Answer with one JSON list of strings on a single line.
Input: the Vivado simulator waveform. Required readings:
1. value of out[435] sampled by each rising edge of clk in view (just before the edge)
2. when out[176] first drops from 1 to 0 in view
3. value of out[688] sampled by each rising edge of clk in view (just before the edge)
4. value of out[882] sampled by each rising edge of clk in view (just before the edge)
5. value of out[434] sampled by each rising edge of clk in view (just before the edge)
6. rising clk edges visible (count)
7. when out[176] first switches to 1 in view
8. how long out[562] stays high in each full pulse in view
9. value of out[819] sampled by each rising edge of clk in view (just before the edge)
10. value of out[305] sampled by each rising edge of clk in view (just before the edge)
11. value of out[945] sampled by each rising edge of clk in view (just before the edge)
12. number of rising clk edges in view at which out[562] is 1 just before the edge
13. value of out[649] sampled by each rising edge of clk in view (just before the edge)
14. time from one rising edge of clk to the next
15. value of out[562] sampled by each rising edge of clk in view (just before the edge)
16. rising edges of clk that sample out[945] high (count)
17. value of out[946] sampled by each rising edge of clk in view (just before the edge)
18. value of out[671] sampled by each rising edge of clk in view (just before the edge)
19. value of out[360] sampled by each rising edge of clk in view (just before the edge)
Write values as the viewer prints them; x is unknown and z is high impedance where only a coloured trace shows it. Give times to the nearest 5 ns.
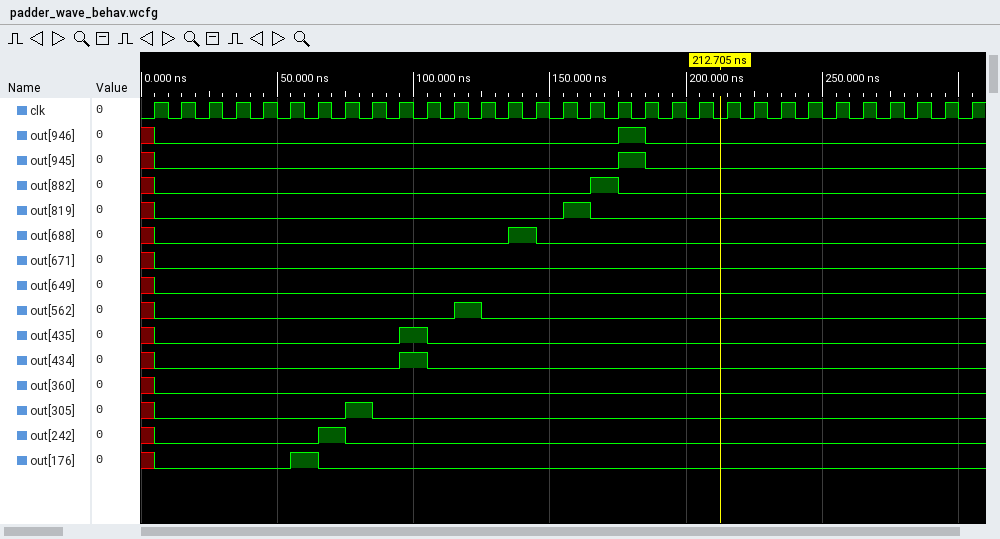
["x 0 0 0 0 0 0 0 0 0 1 0 0 0 0 0 0 0 0 0 0 0 0 0 0 0 0 0 0 0 0", "65 ns", "x 0 0 0 0 0 0 0 0 0 0 0 0 0 1 0 0 0 0 0 0 0 0 0 0 0 0 0 0 0 0", "x 0 0 0 0 0 0 0 0 0 0 0 0 0 0 0 0 1 0 0 0 0 0 0 0 0 0 0 0 0 0", "x 0 0 0 0 0 0 0 0 0 1 0 0 0 0 0 0 0 0 0 0 0 0 0 0 0 0 0 0 0 0", "31", "55 ns", "10 ns", "x 0 0 0 0 0 0 0 0 0 0 0 0 0 0 0 1 0 0 0 0 0 0 0 0 0 0 0 0 0 0", "x 0 0 0 0 0 0 0 1 0 0 0 0 0 0 0 0 0 0 0 0 0 0 0 0 0 0 0 0 0 0", "x 0 0 0 0 0 0 0 0 0 0 0 0 0 0 0 0 0 1 0 0 0 0 0 0 0 0 0 0 0 0", "1", "x 0 0 0 0 0 0 0 0 0 0 0 0 0 0 0 0 0 0 0 0 0 0 0 0 0 0 0 0 0 0", "10 ns", "x 0 0 0 0 0 0 0 0 0 0 0 1 0 0 0 0 0 0 0 0 0 0 0 0 0 0 0 0 0 0", "1", "x 0 0 0 0 0 0 0 0 0 0 0 0 0 0 0 0 0 1 0 0 0 0 0 0 0 0 0 0 0 0", "x 0 0 0 0 0 0 0 0 0 0 0 0 0 0 0 0 0 0 0 0 0 0 0 0 0 0 0 0 0 0", "x 0 0 0 0 0 0 0 0 0 0 0 0 0 0 0 0 0 0 0 0 0 0 0 0 0 0 0 0 0 0"]
